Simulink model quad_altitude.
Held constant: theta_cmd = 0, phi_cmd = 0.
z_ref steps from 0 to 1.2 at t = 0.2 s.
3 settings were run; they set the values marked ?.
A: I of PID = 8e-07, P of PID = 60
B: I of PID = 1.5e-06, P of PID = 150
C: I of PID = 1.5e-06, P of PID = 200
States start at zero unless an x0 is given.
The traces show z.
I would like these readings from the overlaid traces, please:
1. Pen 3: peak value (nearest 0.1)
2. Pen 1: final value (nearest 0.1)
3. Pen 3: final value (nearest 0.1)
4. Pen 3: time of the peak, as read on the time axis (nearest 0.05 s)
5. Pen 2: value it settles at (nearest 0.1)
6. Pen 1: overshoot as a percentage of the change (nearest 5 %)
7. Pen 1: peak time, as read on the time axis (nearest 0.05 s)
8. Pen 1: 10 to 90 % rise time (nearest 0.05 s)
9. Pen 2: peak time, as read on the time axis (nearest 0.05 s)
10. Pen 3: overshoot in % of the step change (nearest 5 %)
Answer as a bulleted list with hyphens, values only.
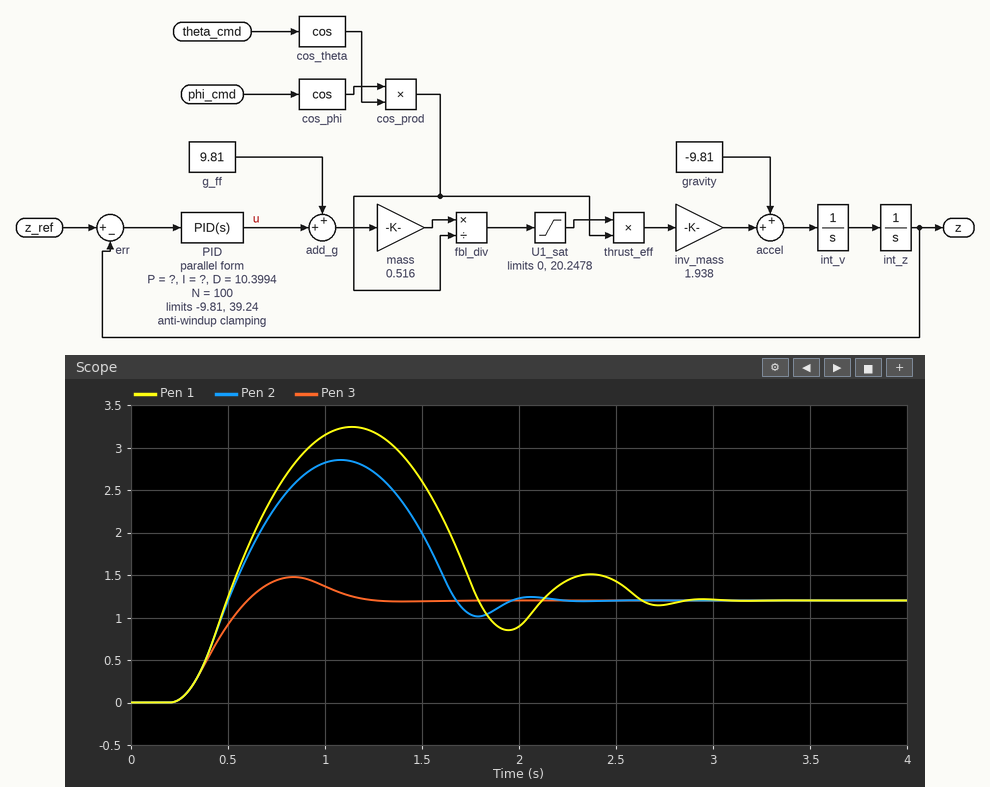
- 1.5
- 1.2
- 1.2
- 0.85 s
- 1.2
- 170 %
- 1.15 s
- 0.20 s
- 1.10 s
- 25 %
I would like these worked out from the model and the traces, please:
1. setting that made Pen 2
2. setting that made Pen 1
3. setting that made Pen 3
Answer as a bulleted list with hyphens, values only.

- B
- C
- A
